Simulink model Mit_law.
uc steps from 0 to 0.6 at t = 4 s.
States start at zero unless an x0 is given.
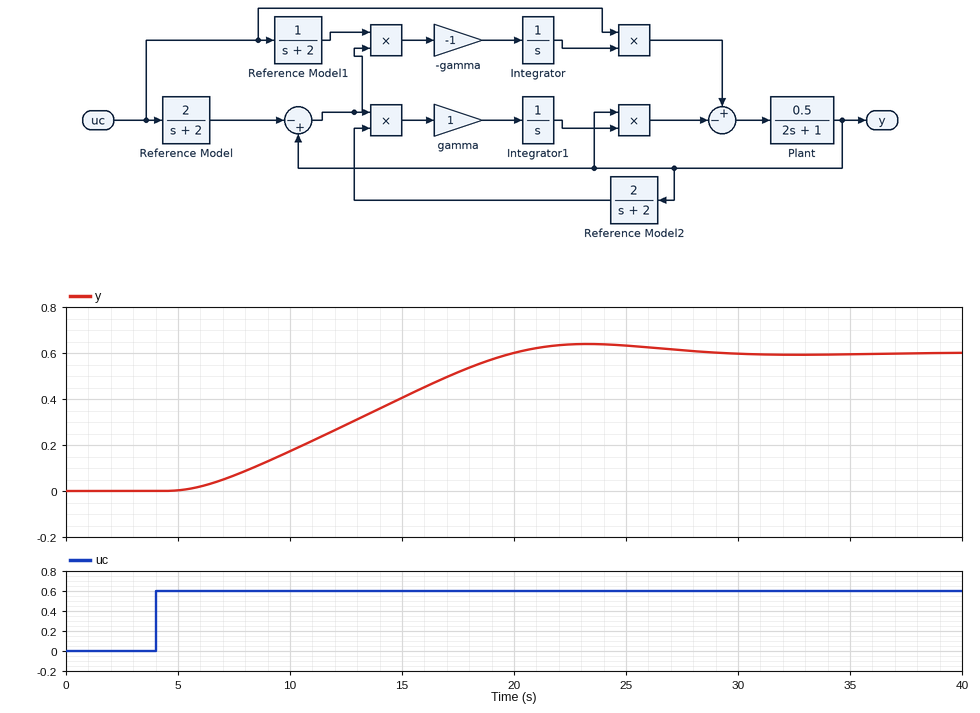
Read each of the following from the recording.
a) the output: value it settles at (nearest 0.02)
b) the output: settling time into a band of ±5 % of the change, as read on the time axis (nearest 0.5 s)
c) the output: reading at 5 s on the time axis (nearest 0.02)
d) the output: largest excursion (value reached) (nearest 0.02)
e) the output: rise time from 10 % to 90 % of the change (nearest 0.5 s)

0.60
25.5 s
0.00
0.64
11.0 s
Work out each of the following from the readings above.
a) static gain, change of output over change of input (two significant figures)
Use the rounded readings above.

1.0
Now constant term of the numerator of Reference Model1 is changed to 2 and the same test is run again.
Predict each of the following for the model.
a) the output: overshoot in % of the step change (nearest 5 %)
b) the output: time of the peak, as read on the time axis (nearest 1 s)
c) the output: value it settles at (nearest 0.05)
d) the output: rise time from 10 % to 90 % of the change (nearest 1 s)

10 %
17 s
0.60
7 s
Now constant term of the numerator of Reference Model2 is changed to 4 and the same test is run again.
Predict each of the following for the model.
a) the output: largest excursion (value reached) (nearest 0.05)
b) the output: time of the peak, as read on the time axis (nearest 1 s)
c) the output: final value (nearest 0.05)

0.70
19 s
0.60
